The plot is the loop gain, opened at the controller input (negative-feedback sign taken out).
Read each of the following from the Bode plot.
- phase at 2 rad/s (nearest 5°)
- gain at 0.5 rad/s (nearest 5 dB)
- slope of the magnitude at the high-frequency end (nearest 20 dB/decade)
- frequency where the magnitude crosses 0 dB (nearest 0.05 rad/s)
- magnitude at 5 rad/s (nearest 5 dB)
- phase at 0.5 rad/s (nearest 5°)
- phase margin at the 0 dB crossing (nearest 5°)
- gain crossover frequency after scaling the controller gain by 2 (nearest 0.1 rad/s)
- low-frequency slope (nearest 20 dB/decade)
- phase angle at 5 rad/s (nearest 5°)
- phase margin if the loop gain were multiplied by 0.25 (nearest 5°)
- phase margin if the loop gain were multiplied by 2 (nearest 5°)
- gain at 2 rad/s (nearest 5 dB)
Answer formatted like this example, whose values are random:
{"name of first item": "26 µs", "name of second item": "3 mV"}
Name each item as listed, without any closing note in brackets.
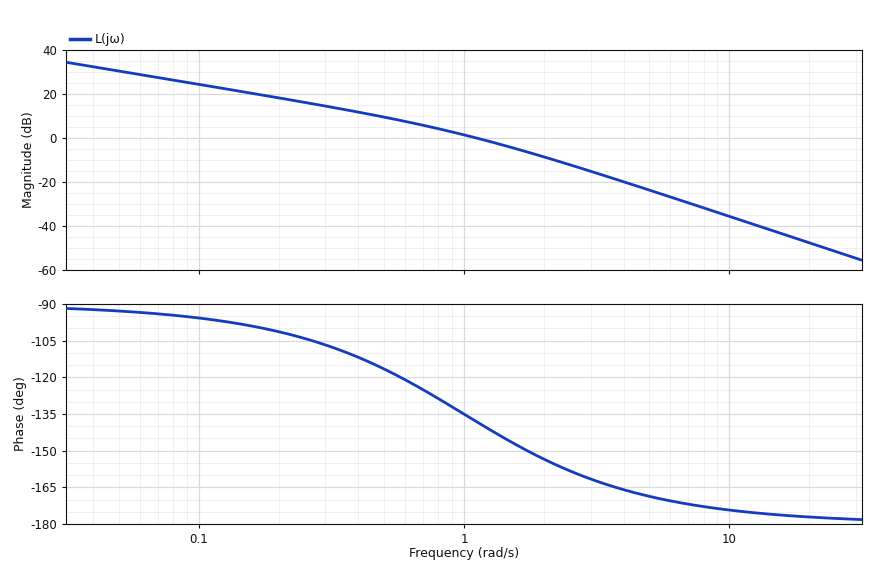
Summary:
{"phase at 2 rad/s": "-155°", "gain at 0.5 rad/s": "10 dB", "slope of the magnitude at the high-frequency end": "-40 dB/decade", "frequency where the magnitude crosses 0 dB": "1.10 rad/s", "magnitude at 5 rad/s": "-25 dB", "phase at 0.5 rad/s": "-115°", "phase margin at the 0 dB crossing": "40°", "gain crossover frequency after scaling the controller gain by 2": "1.7 rad/s", "low-frequency slope": "-20 dB/decade", "phase angle at 5 rad/s": "-170°", "phase margin if the loop gain were multiplied by 0.25": "70°", "phase margin if the loop gain were multiplied by 2": "30°", "gain at 2 rad/s": "-10 dB"}
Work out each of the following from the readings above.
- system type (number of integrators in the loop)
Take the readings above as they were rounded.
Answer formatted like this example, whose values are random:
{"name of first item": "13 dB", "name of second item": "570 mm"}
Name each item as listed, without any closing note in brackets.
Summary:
{"system type": "1"}
